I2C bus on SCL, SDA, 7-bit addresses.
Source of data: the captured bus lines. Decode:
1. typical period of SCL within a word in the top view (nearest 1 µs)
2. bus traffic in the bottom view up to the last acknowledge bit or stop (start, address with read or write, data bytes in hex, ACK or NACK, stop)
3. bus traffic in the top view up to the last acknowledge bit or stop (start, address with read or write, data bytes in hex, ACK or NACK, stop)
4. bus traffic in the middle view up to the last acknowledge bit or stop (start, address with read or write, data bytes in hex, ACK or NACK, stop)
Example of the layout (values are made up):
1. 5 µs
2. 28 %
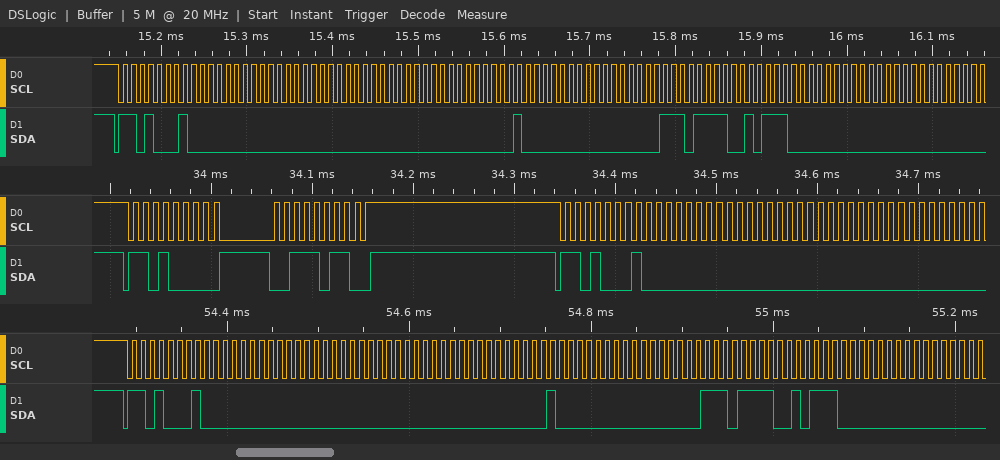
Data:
1. 10 µs
2. start, address 68 read ACK, 00 ACK, 00 ACK, 00 ACK, 00 ACK, 40 ACK, 00 ACK, EF ACK, 5C ACK, 00 ACK
3. start, address 68 read ACK, 00 ACK, 00 ACK, 00 ACK, 00 ACK, 40 ACK, 00 ACK, EF ACK, 5C ACK, 00 ACK, 00 ACK
4. start, address 68 write ACK, 3B ACK, stop, start, address 68 read ACK, 00 ACK, 00 ACK, 00 ACK
